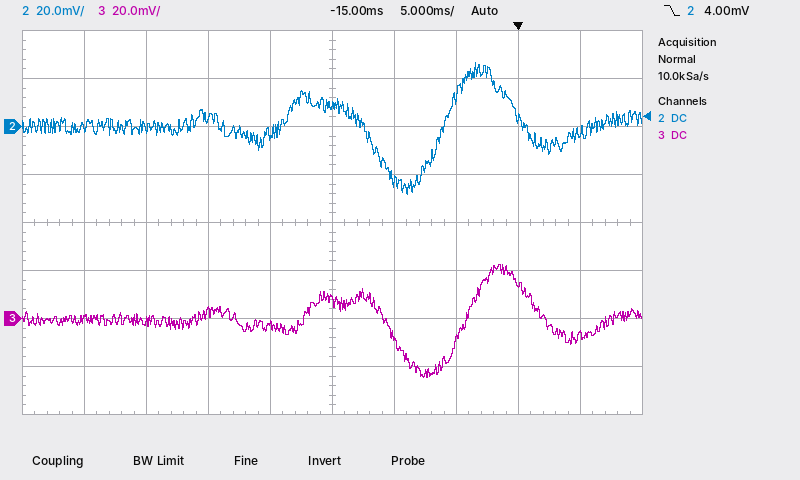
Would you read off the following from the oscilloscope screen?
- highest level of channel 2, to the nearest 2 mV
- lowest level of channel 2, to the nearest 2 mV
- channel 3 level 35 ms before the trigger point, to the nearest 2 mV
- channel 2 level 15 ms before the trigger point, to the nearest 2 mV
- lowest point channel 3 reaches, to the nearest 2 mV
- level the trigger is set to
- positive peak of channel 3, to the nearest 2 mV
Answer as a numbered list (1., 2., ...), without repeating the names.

1. 26 mV
2. -28 mV
3. 0 mV
4. 8 mV
5. -24 mV
6. 4.00 mV
7. 22 mV
